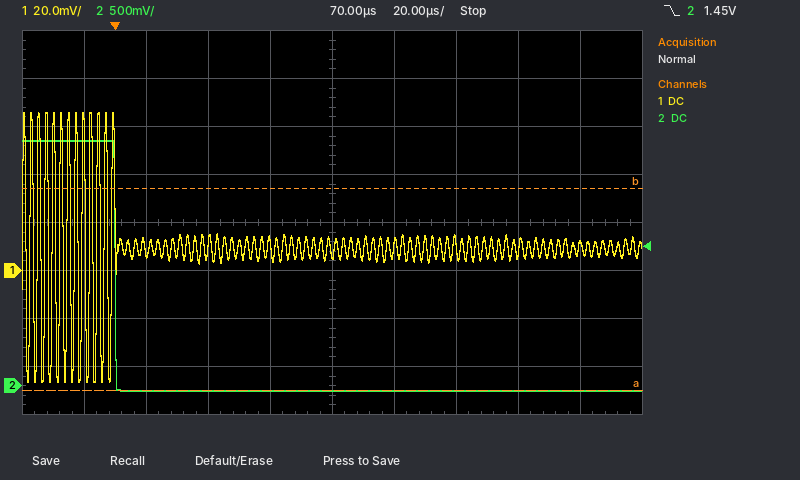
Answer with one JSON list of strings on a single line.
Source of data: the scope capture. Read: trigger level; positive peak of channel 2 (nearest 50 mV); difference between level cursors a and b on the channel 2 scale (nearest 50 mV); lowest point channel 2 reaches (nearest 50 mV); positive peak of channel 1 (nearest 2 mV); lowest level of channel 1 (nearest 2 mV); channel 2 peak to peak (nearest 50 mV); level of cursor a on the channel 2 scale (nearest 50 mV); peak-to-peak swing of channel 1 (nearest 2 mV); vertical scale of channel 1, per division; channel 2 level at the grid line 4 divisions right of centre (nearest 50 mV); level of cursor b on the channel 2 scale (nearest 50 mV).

["1.45 V", "2.55 V", "2.10 V", "-50 mV", "66 mV", "-46 mV", "2.60 V", "-50 mV", "112 mV", "20 mV", "-50 mV", "2.05 V"]
